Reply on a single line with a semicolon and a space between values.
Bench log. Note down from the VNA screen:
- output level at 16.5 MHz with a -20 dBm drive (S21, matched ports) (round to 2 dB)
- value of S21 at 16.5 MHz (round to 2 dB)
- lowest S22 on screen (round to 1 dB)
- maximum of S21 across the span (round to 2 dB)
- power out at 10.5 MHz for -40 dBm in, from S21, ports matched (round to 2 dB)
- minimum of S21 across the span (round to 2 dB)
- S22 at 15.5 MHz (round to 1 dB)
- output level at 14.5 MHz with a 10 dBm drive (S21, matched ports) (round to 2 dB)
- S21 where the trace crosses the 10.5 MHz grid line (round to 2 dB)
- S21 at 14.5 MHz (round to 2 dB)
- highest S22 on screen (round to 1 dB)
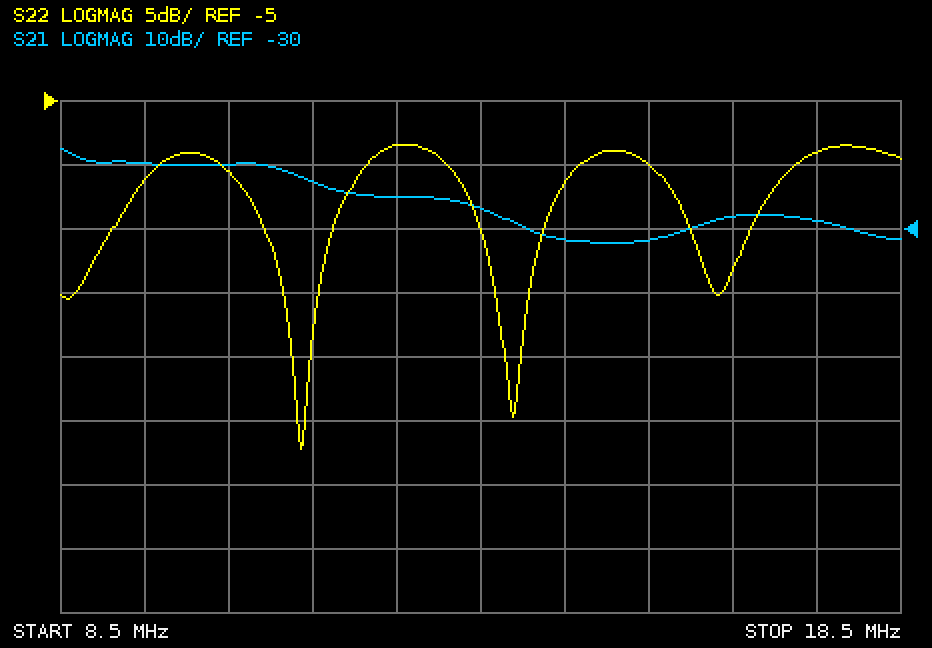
-48 dBm; -28 dB; -32 dB; -18 dB; -60 dBm; -32 dB; -10 dB; -22 dBm; -20 dB; -32 dB; -8 dB
